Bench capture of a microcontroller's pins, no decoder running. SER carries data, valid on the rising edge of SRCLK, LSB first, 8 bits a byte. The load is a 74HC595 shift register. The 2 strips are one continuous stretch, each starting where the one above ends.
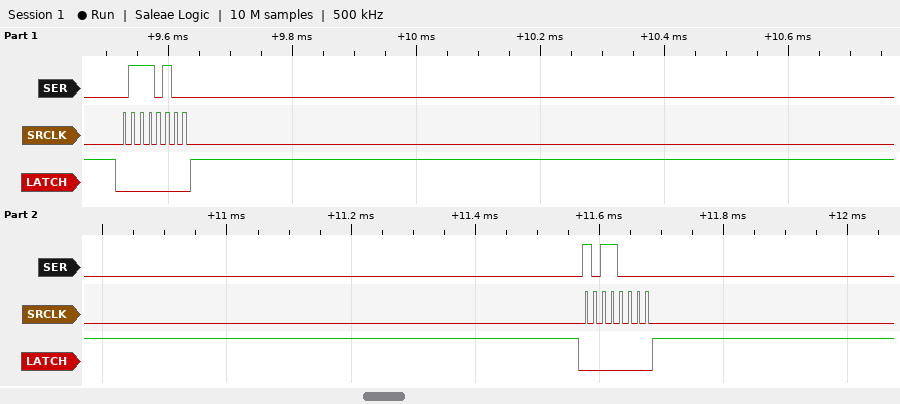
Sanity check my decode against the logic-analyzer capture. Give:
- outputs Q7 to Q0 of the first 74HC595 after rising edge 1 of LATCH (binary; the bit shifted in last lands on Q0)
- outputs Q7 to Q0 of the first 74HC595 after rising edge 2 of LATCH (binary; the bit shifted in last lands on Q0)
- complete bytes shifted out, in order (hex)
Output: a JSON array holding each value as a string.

["01110100", "10110000", "2E 0D"]
